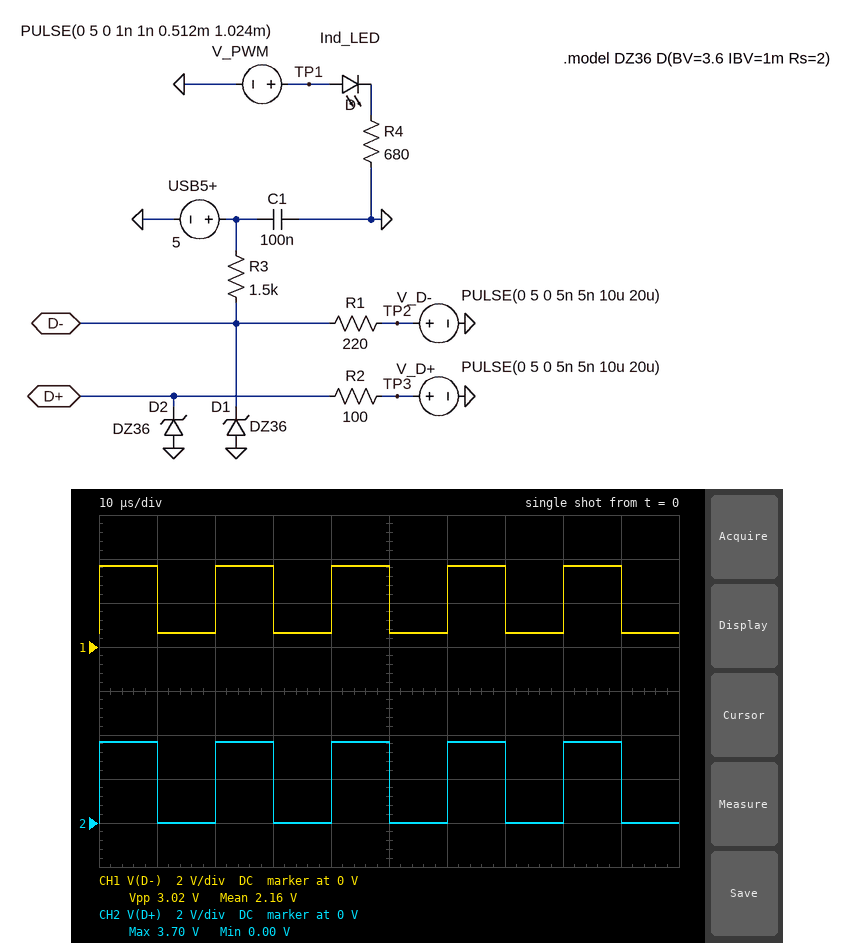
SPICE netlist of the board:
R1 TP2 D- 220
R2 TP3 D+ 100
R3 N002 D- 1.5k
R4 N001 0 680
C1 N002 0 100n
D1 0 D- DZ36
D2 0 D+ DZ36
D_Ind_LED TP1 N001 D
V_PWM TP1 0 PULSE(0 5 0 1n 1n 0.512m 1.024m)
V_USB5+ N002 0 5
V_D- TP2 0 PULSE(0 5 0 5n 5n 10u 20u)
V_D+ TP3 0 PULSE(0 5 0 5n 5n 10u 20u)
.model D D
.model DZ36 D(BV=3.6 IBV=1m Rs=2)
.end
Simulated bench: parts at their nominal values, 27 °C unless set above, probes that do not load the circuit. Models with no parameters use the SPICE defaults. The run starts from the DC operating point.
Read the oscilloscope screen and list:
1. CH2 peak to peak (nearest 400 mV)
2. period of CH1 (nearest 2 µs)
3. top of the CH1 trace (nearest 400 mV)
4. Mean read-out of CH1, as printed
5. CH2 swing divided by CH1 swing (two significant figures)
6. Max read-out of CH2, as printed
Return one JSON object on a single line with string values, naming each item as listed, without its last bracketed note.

{"CH2 peak to peak": "3.6 V", "period of CH1": "20 µs", "top of the CH1 trace": "3.6 V", "Mean read-out of CH1, as printed": "2.16 V", "CH2 swing divided by CH1 swing": "1.2", "Max read-out of CH2, as printed": "3.70 V"}
